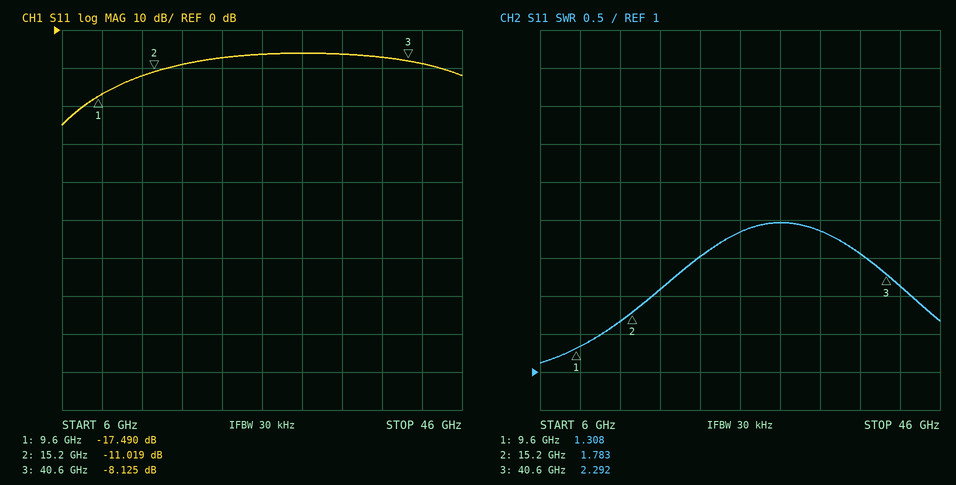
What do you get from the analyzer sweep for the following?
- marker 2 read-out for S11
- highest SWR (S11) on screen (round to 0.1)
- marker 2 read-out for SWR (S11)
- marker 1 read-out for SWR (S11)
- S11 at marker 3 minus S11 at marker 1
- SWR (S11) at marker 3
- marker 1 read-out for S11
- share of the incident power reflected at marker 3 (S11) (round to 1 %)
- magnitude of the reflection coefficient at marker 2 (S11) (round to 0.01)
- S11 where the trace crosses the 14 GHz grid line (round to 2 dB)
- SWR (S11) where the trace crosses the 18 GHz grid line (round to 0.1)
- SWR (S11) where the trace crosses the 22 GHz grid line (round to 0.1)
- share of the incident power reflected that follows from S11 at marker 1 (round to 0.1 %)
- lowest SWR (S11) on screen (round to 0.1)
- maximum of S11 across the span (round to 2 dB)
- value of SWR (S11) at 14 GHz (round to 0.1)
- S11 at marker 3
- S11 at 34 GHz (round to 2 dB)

-11.019 dB
3.0
1.783
1.308
9.365 dB
2.292
-17.490 dB
15 %
0.28
-12 dB
2.1
2.5
1.8 %
1.1
-6 dB
1.7
-8.125 dB
-6 dB
